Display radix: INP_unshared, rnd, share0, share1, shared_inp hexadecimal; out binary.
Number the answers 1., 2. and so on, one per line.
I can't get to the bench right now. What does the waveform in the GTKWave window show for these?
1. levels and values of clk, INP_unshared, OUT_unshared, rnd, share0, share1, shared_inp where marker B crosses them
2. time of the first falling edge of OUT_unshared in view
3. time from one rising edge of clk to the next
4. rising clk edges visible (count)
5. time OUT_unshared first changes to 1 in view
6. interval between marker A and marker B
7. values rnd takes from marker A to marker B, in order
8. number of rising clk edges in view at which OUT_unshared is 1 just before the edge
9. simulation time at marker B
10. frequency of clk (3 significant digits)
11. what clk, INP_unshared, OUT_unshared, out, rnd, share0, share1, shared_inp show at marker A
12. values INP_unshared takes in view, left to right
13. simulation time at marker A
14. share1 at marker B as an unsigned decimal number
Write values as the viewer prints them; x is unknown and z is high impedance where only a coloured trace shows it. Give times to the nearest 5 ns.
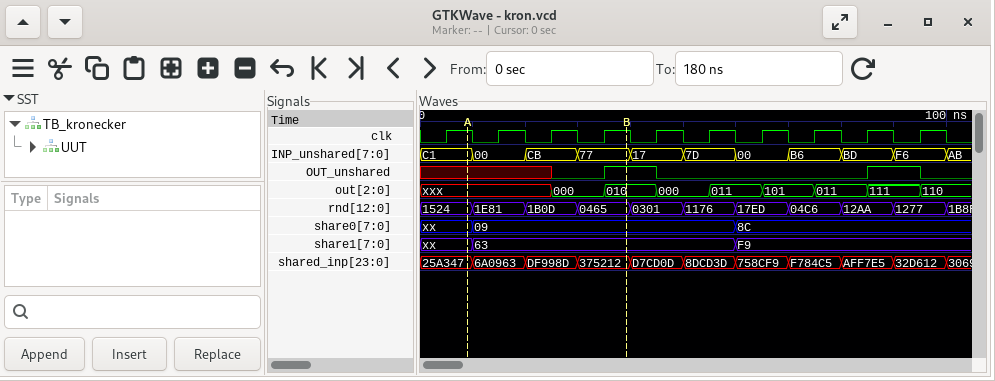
1. clk=1, INP_unshared=77, OUT_unshared=1, rnd=0465, share0=09, share1=63, shared_inp=375212
2. 45 ns
3. 10 ns
4. 10
5. 35 ns
6. 30 ns
7. 1524, 1E81, 1B0D, 0465
8. 2
9. 40 ns
10. 100 MHz
11. clk=1, INP_unshared=C1, OUT_unshared=x, out=xxx, rnd=1524, share0=xx, share1=xx, shared_inp=25A347
12. C1, 00, CB, 77, 17, 7D, 00, B6, BD, F6, AB
13. 10 ns
14. 99
